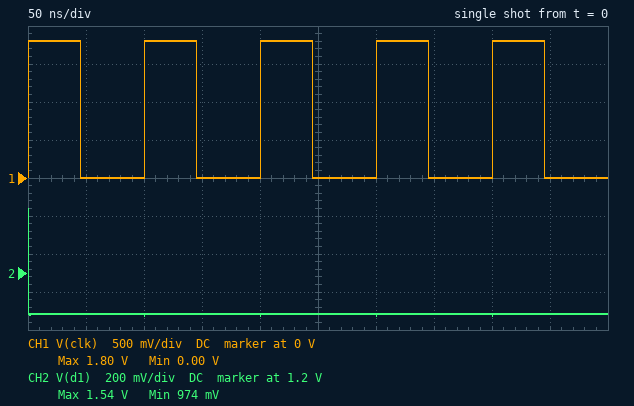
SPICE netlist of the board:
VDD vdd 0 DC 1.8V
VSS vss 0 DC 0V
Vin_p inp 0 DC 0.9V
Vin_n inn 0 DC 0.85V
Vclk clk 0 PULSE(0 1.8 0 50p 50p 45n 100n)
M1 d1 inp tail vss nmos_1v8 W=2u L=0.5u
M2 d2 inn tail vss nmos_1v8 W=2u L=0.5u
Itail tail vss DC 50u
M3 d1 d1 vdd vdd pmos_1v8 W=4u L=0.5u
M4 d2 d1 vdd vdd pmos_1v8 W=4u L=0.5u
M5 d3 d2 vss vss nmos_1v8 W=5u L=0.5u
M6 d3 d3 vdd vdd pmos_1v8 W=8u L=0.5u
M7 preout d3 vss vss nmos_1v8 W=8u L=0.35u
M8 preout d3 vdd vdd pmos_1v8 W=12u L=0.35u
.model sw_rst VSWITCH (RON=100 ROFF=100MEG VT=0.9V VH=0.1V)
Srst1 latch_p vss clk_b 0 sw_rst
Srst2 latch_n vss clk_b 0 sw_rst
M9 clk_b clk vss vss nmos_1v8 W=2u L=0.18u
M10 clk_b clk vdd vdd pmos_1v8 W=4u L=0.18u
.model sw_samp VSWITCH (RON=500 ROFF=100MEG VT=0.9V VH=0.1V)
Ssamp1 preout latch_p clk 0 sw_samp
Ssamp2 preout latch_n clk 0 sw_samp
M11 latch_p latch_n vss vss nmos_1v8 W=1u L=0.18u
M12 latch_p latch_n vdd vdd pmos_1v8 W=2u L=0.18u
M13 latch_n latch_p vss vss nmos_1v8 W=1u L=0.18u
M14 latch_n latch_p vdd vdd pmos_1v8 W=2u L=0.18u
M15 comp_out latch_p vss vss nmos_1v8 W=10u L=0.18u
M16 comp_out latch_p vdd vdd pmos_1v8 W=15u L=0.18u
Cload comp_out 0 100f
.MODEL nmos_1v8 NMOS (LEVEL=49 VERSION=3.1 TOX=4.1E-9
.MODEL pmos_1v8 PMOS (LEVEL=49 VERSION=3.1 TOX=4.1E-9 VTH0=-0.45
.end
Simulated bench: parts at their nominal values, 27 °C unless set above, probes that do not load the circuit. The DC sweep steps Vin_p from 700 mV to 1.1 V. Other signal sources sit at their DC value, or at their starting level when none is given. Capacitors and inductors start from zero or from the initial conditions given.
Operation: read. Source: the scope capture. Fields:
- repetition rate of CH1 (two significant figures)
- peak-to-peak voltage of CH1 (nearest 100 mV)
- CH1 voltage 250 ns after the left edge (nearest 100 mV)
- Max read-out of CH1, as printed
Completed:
10 MHz
1.8 V
0 V
1.80 V
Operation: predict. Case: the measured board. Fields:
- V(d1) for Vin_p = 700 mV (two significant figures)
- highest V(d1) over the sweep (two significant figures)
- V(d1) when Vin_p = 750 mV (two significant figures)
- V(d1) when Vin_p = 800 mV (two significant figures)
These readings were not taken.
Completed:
1.0 V
1.0 V
1.0 V
1.0 V
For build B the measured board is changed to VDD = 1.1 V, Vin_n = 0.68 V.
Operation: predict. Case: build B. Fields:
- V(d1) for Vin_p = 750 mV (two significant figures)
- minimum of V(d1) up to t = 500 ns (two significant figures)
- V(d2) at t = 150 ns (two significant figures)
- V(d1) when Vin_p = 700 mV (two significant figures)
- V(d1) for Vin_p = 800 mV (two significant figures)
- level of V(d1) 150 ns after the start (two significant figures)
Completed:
280 mV
230 mV
1.1 V
300 mV
260 mV
240 mV
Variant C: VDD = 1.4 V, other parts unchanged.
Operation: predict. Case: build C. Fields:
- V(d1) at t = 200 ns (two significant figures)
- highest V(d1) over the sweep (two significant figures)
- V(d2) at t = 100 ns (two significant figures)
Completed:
580 mV
610 mV
1.3 V
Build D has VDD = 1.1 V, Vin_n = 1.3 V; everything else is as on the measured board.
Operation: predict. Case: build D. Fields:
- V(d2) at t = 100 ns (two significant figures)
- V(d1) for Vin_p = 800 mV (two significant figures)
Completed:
220 mV
310 mV
